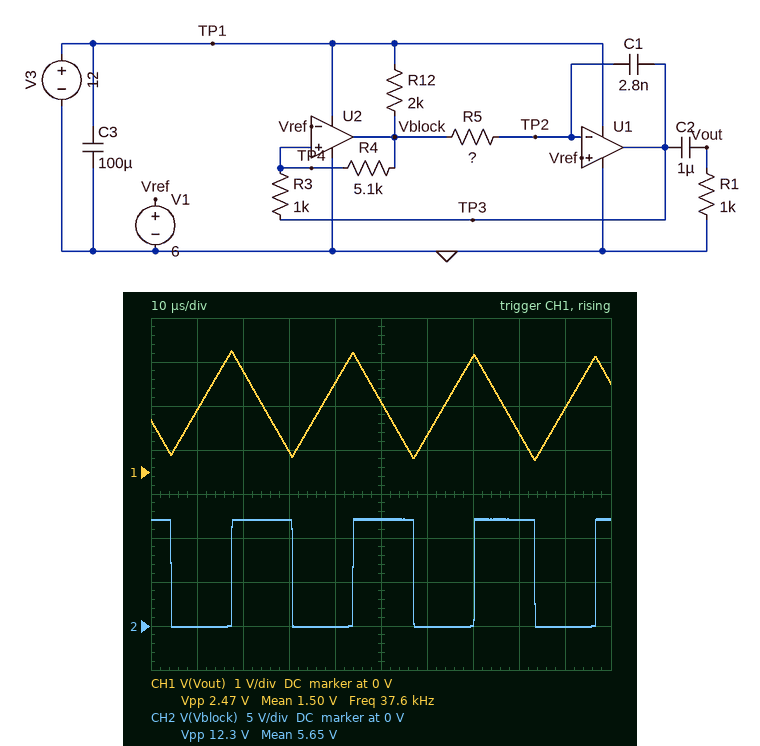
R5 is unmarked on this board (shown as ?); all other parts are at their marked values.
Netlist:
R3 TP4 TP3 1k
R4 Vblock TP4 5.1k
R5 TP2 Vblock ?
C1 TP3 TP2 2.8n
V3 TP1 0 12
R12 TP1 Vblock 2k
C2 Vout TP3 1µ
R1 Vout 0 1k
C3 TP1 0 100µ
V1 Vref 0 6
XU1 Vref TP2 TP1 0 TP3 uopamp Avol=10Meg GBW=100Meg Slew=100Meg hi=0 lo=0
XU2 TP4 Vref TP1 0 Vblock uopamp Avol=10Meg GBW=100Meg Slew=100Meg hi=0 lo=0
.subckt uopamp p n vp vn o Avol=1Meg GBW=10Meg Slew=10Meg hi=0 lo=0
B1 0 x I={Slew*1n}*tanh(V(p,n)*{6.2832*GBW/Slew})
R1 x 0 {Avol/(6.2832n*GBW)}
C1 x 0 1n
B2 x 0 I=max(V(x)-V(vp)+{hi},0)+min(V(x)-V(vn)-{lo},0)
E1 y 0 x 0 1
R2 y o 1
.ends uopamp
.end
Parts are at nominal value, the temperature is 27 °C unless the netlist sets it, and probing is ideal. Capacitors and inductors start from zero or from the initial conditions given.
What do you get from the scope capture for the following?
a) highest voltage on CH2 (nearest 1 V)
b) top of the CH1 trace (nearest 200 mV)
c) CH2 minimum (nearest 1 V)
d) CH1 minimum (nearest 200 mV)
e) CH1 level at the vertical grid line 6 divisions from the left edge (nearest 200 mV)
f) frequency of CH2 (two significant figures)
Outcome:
12 V
2.8 V
0 V
200 mV
800 mV
38 kHz
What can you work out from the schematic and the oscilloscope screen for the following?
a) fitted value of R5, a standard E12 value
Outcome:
12 kΩ
